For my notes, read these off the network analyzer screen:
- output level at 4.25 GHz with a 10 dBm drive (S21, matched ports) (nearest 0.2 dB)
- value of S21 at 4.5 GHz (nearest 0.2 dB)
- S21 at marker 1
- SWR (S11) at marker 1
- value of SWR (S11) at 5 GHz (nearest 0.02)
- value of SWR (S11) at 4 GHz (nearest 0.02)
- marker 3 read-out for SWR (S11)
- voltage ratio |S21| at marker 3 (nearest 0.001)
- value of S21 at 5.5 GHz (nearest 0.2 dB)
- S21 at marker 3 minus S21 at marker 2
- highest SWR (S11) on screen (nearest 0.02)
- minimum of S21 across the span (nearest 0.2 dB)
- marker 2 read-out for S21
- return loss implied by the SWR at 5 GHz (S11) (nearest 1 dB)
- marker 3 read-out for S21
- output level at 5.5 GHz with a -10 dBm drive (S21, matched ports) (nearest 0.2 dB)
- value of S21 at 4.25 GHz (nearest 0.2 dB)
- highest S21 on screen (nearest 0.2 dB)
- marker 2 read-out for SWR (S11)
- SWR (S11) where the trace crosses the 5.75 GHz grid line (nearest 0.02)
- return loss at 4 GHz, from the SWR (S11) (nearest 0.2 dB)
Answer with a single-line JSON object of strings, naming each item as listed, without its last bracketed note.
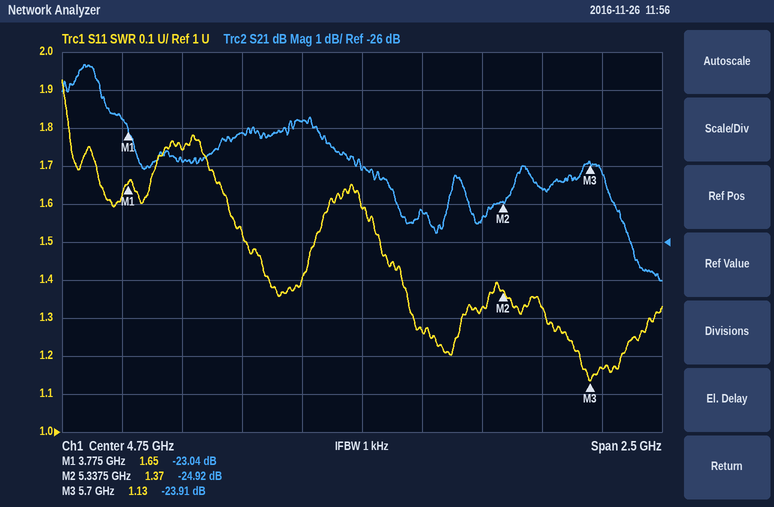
{"output level at 4.25 GHz with a 10 dBm drive (S21, matched ports)": "-13.2 dBm", "value of S21 at 4.5 GHz": "-22.8 dB", "S21 at marker 1": "-23.04 dB", "SWR (S11) at marker 1": "1.65", "value of SWR (S11) at 5 GHz": "1.26", "value of SWR (S11) at 4 GHz": "1.74", "marker 3 read-out for SWR": "1.13", "voltage ratio |S21| at marker 3": "0.064", "value of S21 at 5.5 GHz": "-24.6 dB", "S21 at marker 3 minus S21 at marker 2": "1.01 dB", "highest SWR (S11) on screen": "1.92", "minimum of S21 across the span": "-27.0 dB", "marker 2 read-out for S21": "-24.92 dB", "return loss implied by the SWR at 5 GHz (S11)": "19 dB", "marker 3 read-out for S21": "-23.91 dB", "output level at 5.5 GHz with a -10 dBm drive (S21, matched ports)": "-34.6 dBm", "value of S21 at 4.25 GHz": "-23.2 dB", "highest S21 on screen": "-21.4 dB", "marker 2 read-out for SWR": "1.37", "SWR (S11) where the trace crosses the 5.75 GHz grid line": "1.16", "return loss at 4 GHz, from the SWR (S11)": "11.4 dB"}
